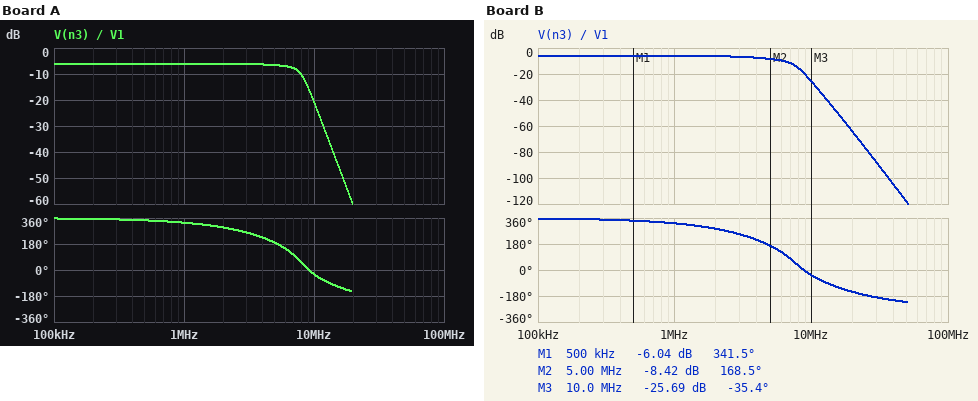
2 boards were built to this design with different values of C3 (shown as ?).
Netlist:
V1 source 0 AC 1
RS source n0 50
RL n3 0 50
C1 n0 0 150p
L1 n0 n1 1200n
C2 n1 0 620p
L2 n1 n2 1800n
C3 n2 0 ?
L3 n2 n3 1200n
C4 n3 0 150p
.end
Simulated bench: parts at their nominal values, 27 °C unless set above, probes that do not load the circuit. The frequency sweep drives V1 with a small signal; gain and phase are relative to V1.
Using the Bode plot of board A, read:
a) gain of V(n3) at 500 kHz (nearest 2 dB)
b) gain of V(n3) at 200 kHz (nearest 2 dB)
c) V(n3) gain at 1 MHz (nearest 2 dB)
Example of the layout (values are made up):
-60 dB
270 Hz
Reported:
-6 dB
-6 dB
-6 dB
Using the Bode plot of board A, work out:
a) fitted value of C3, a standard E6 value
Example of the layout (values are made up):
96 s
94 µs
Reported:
1 nF
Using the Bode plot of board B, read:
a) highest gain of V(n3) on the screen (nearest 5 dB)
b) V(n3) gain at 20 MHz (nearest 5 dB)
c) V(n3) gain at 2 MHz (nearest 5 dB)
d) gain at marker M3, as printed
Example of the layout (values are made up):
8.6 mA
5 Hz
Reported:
-5 dB
-65 dB
-5 dB
-25.69 dB
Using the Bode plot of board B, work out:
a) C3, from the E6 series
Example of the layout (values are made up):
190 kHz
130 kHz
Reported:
1.5 nF
